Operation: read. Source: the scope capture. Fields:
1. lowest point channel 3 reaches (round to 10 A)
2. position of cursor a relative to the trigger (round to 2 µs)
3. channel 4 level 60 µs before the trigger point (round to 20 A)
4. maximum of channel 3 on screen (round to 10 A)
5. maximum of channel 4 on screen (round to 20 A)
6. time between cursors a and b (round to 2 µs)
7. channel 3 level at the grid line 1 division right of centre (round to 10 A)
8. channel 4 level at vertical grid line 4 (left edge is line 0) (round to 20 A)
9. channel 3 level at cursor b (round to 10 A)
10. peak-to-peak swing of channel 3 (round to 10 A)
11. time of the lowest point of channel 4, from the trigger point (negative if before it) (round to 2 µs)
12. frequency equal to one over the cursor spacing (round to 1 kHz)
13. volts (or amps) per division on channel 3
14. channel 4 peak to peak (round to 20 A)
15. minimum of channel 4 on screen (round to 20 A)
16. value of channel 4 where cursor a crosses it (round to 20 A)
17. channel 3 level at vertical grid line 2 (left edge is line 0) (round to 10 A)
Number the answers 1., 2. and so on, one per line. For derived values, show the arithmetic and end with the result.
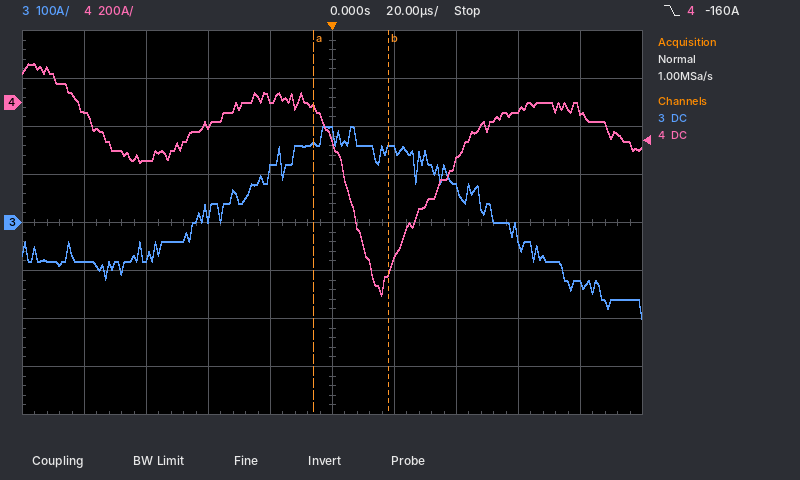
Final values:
1. -200 A
2. -6 µs
3. -240 A
4. 200 A
5. 160 A
6. 24 µs
7. 150 A
8. 20 A
9. 150 A
10. 200 A − (-200 A) = 400 A
11. +16 µs
12. 1 / 24 µs ≈ 42 kHz
13. 100 A
14. 160 A − (-800 A) = 960 A
15. -800 A
16. -20 A
17. -70 A
